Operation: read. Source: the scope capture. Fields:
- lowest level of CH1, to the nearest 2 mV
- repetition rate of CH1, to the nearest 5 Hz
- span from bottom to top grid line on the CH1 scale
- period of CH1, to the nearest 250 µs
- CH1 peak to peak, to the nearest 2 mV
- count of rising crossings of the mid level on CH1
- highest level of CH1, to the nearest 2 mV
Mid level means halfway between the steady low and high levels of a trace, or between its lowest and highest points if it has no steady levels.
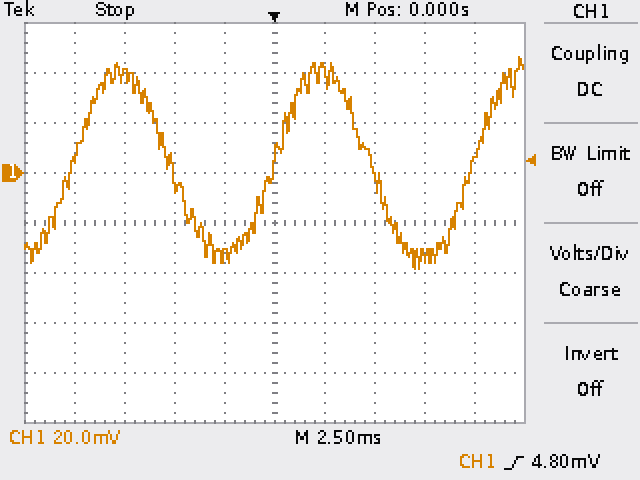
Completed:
-38 mV
100 Hz
160 mV
10.00 ms
84 mV
3
46 mV
